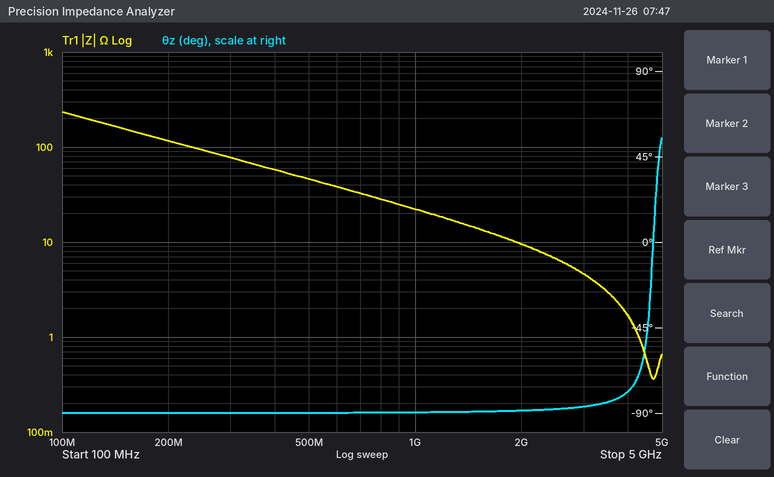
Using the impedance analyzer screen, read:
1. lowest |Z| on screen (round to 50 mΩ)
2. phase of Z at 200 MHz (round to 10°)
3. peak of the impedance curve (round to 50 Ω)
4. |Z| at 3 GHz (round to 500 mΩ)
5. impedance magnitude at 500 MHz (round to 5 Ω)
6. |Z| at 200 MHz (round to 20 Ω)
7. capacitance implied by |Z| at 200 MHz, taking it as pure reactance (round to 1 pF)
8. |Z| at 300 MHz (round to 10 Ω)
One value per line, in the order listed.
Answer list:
350 mΩ
-90°
250 Ω
4.5 Ω
45 Ω
120 Ω
7 pF
80 Ω
